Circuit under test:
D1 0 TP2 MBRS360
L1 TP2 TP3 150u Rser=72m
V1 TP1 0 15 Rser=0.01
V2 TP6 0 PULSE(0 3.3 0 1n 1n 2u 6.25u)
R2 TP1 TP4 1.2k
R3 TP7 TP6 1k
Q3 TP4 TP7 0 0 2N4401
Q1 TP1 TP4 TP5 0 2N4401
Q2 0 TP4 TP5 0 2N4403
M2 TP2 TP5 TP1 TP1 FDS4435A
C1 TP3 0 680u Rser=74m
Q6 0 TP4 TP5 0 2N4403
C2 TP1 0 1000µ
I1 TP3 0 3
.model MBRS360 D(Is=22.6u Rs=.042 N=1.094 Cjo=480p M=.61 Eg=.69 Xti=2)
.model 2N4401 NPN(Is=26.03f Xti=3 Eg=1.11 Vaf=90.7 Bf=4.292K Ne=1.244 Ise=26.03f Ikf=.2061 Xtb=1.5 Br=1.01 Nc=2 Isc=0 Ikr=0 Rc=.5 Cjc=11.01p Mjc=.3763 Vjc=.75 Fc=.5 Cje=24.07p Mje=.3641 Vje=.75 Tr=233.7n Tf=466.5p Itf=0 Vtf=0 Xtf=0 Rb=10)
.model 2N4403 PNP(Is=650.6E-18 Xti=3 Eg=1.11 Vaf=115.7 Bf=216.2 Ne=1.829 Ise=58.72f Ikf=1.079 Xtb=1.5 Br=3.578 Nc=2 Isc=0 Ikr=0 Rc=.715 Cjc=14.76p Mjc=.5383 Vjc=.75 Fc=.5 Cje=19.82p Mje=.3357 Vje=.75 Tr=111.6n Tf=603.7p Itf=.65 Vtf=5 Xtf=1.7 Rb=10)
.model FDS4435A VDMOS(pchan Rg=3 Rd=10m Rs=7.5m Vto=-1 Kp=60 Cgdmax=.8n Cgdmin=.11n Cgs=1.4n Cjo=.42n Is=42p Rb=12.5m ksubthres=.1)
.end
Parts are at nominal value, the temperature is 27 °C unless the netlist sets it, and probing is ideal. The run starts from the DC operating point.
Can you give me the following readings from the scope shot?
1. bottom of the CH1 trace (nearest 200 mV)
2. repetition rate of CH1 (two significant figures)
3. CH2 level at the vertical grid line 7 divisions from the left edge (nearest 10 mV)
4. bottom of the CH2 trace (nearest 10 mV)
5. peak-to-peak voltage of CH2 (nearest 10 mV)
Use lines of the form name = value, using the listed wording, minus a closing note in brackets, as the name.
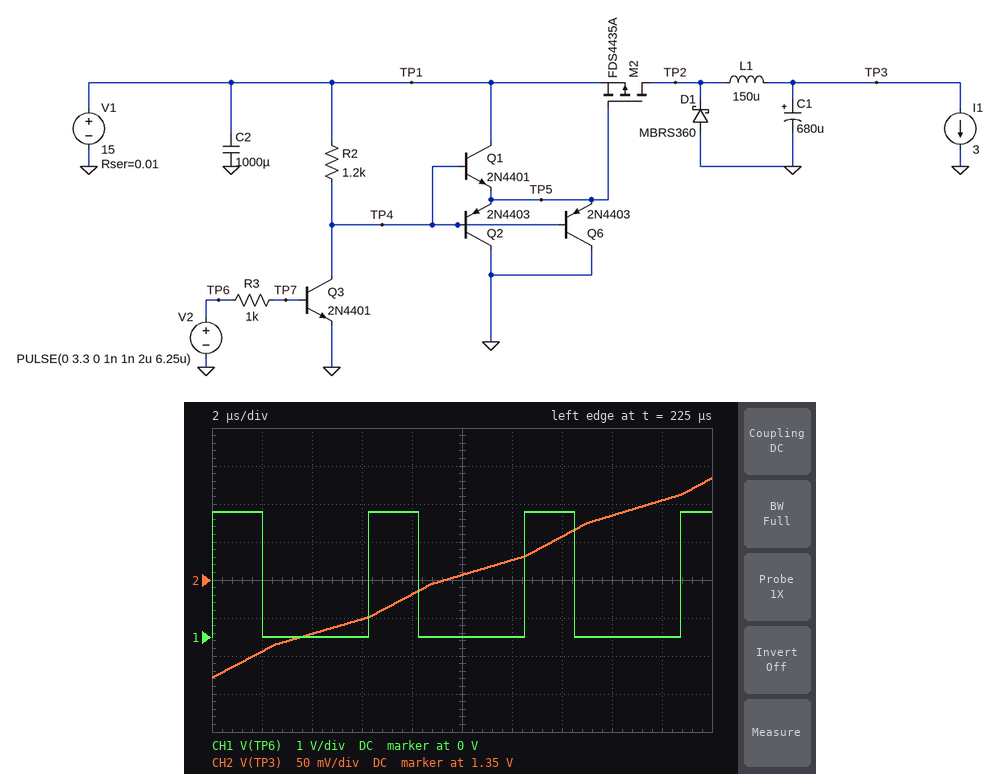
bottom of the CH1 trace = 0 V
repetition rate of CH1 = 160 kHz
CH2 level at the vertical grid line 7 divisions from the left edge = 1.41 V
bottom of the CH2 trace = 1.22 V
peak-to-peak voltage of CH2 = 260 mV
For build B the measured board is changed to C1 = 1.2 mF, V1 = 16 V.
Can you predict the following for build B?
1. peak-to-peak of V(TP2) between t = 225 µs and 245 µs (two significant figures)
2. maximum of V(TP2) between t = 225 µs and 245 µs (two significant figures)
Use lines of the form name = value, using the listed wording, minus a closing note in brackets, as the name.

peak-to-peak of V(TP2) between t = 225 µs and 245 µs = 17 V
maximum of V(TP2) between t = 225 µs and 245 µs = 16 V
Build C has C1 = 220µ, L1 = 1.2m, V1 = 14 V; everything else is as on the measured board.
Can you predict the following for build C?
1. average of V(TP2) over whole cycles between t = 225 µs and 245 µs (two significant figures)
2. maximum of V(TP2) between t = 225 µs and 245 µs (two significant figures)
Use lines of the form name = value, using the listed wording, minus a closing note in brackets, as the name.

average of V(TP2) over whole cycles between t = 225 µs and 245 µs = 5.2 V
maximum of V(TP2) between t = 225 µs and 245 µs = 14 V
